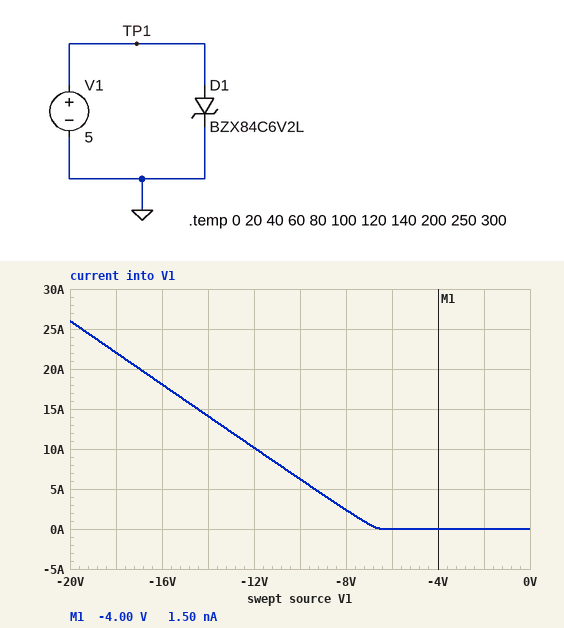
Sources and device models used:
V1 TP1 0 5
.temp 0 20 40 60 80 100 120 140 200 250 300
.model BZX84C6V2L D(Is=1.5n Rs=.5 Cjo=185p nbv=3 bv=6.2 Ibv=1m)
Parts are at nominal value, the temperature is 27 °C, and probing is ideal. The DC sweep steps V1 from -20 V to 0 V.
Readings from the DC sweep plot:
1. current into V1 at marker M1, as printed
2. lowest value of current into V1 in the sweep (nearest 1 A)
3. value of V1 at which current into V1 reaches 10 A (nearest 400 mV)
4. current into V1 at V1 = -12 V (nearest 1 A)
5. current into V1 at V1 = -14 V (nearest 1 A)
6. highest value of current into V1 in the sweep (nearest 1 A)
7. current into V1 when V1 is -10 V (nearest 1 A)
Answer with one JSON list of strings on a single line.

["1.50 nA", "0 A", "-12.0 V", "10 A", "14 A", "26 A", "6 A"]
